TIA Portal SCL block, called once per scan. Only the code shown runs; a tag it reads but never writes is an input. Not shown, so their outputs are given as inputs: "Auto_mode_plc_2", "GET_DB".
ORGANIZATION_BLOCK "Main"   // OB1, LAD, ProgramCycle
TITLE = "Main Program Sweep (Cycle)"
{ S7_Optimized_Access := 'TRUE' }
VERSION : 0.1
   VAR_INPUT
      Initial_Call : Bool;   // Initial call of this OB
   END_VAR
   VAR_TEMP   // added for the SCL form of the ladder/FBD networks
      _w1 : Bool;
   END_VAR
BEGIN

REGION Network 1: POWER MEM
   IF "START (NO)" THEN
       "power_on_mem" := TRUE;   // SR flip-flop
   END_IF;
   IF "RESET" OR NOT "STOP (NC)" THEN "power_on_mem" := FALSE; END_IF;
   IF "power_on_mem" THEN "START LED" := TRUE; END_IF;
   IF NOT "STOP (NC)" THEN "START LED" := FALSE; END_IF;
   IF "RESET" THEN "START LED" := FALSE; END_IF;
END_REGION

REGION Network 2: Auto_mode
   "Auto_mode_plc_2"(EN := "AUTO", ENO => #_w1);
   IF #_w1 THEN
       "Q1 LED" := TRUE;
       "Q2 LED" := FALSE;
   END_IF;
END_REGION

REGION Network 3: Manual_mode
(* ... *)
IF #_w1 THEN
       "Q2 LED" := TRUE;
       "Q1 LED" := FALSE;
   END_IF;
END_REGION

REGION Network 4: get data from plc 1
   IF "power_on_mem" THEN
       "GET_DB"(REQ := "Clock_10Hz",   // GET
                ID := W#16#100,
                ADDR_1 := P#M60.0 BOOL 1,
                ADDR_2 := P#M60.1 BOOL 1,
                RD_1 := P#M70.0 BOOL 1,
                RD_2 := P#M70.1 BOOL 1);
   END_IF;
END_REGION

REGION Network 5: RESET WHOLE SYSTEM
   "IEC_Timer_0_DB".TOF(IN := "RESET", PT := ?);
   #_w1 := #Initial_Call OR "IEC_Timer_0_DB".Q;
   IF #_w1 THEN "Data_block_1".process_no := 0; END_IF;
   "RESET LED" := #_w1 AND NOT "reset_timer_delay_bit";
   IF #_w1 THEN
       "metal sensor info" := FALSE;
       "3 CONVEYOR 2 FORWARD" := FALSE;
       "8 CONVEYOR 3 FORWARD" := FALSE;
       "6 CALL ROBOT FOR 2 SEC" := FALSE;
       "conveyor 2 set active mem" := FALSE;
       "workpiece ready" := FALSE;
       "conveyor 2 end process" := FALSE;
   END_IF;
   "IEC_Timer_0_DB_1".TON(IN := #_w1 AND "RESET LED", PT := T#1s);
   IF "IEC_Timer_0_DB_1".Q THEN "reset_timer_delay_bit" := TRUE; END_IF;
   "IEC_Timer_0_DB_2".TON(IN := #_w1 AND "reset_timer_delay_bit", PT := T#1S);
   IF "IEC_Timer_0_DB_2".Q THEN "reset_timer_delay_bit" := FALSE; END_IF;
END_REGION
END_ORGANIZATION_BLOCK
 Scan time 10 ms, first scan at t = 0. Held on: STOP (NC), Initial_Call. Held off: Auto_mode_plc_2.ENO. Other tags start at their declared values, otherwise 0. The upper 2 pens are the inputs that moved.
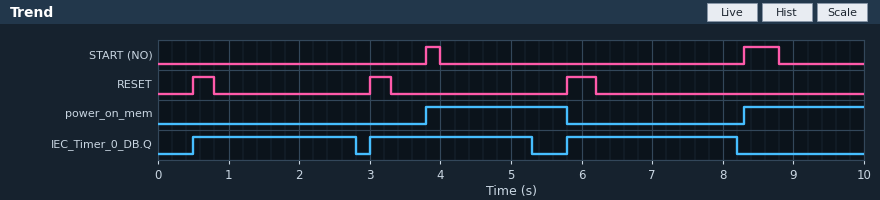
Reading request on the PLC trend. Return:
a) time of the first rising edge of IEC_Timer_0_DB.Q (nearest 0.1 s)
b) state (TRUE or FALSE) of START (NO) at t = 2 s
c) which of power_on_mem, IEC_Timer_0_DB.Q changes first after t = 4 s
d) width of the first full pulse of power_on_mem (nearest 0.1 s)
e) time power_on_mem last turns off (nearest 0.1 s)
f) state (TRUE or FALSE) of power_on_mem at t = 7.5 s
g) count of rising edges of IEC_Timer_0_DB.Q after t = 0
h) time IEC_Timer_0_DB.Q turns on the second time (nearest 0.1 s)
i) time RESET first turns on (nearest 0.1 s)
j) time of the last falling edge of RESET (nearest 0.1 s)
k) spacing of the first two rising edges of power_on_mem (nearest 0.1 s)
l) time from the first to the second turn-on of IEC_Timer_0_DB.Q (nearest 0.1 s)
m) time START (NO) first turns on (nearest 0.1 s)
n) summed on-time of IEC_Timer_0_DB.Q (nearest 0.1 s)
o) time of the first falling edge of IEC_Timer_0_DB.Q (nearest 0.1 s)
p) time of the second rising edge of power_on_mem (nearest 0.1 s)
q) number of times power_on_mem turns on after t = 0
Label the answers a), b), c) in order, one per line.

a) 0.5 s
b) FALSE
c) IEC_Timer_0_DB.Q
d) 2.0 s
e) 5.8 s
f) FALSE
g) 3
h) 3.0 s
i) 0.5 s
j) 6.2 s
k) 4.5 s
l) 2.5 s
m) 3.8 s
n) 7.0 s
o) 2.8 s
p) 8.3 s
q) 2
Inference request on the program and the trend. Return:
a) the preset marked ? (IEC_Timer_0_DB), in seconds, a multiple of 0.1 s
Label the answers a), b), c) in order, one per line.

a) 2.0 s
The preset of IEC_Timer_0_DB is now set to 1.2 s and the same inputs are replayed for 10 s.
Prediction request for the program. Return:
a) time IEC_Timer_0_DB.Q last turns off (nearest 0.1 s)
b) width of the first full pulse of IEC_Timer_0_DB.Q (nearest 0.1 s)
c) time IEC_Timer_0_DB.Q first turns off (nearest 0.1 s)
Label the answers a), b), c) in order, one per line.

a) 7.4 s
b) 1.5 s
c) 2.0 s
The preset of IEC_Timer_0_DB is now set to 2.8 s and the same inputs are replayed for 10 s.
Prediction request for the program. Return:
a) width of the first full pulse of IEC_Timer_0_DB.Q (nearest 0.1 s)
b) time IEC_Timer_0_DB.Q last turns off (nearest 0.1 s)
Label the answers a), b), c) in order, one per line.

a) 8.5 s
b) 9.0 s
